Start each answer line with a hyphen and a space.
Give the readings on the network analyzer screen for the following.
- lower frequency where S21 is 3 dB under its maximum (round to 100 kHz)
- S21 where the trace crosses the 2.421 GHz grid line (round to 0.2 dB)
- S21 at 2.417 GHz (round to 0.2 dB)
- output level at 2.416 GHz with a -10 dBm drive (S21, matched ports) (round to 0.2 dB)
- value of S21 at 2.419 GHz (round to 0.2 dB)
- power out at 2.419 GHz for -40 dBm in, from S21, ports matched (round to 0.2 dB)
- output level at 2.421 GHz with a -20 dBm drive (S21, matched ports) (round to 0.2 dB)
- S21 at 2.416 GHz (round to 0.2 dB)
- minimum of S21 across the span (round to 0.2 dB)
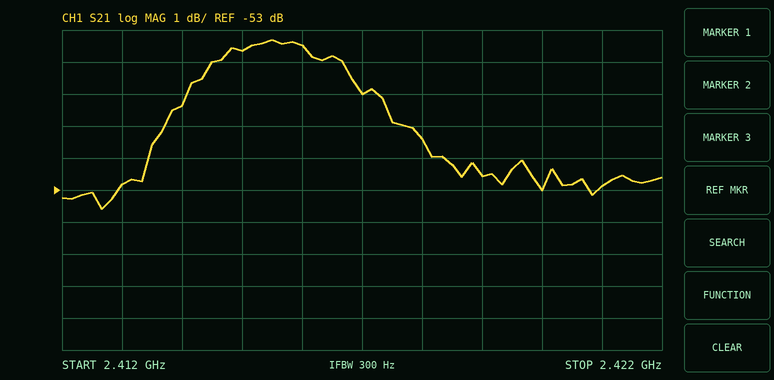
- 2.4136 GHz
- -52.8 dB
- -50.0 dB
- -58.4 dBm
- -52.6 dB
- -92.6 dBm
- -72.8 dBm
- -48.4 dB
- -53.6 dB
